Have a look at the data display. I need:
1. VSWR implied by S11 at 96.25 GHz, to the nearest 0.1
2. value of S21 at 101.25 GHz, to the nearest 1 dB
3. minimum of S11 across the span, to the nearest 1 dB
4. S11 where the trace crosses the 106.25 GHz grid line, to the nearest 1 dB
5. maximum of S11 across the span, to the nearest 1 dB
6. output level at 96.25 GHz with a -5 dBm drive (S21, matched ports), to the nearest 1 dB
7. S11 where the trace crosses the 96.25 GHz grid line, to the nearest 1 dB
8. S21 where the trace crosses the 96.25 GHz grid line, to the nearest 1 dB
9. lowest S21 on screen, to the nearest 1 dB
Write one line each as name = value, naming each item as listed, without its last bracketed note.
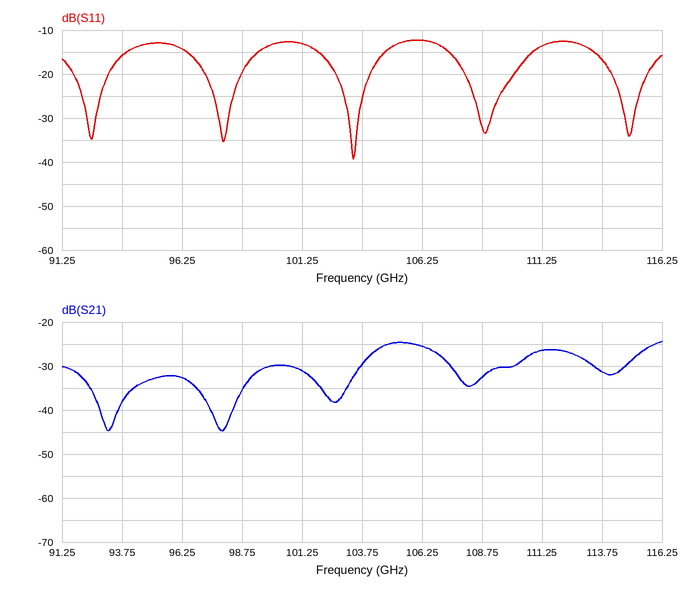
VSWR implied by S11 at 96.25 GHz, to the nearest 0.1 = 1.5
value of S21 at 101.25 GHz, to the nearest 1 dB = -31 dB
minimum of S11 across the span, to the nearest 1 dB = -39 dB
S11 where the trace crosses the 106.25 GHz grid line, to the nearest 1 dB = -12 dB
maximum of S11 across the span, to the nearest 1 dB = -12 dB
output level at 96.25 GHz with a -5 dBm drive (S21, matched ports), to the nearest 1 dB = -38 dBm
S11 where the trace crosses the 96.25 GHz grid line, to the nearest 1 dB = -14 dB
S21 where the trace crosses the 96.25 GHz grid line, to the nearest 1 dB = -33 dB
lowest S21 on screen, to the nearest 1 dB = -45 dB
